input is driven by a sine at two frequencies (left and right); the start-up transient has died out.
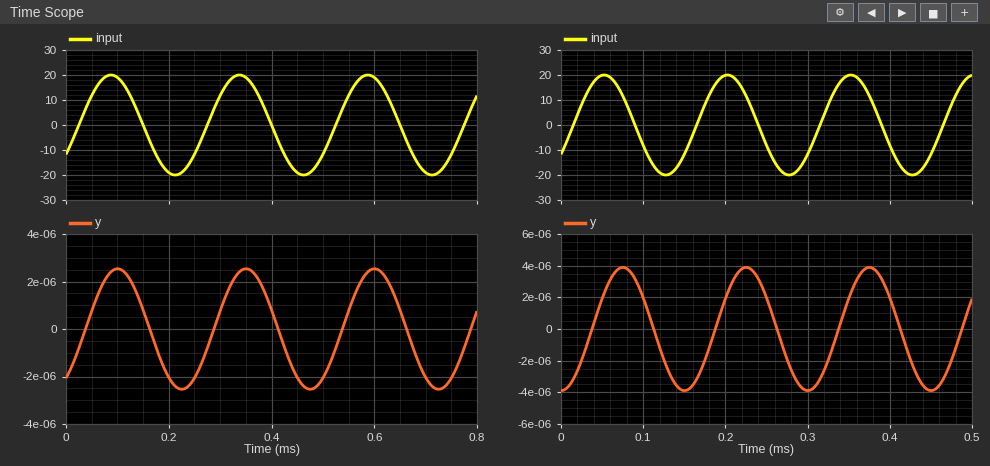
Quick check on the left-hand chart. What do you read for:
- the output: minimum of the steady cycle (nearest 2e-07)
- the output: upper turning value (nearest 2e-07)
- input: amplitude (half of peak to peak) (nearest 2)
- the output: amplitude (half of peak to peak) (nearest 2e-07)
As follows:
-0.0000026
0.0000026
20
0.0000026
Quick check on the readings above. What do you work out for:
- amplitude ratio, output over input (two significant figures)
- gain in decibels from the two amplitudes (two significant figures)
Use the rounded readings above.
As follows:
0.00000013
-140 dB
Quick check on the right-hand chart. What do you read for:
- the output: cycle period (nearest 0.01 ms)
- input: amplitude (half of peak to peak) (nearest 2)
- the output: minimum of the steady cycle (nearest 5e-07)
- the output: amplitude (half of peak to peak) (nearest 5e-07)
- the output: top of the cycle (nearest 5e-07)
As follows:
0.15 ms
20
-0.0000040
0.0000040
0.0000040
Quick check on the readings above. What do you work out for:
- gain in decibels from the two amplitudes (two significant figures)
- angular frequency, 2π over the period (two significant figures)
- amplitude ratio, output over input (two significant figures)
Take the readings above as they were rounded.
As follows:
-130 dB
42 rad/ms
0.00000020
